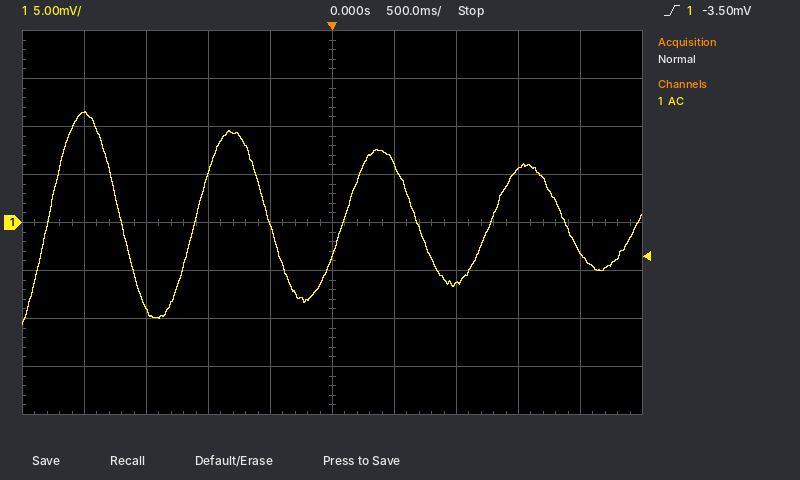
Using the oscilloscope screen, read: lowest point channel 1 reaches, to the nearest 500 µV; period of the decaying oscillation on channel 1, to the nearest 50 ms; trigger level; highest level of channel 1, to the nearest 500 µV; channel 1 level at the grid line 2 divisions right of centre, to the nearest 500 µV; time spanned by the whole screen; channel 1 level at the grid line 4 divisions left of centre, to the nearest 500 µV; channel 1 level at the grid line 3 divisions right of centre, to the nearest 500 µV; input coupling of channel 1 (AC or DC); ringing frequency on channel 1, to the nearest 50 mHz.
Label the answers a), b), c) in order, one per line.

a) -10.5 mV
b) 1.20 s
c) -3.50 mV
d) 11.5 mV
e) -6.5 mV
f) 5 s
g) 11.5 mV
h) 5.5 mV
i) AC
j) 850 mHz
